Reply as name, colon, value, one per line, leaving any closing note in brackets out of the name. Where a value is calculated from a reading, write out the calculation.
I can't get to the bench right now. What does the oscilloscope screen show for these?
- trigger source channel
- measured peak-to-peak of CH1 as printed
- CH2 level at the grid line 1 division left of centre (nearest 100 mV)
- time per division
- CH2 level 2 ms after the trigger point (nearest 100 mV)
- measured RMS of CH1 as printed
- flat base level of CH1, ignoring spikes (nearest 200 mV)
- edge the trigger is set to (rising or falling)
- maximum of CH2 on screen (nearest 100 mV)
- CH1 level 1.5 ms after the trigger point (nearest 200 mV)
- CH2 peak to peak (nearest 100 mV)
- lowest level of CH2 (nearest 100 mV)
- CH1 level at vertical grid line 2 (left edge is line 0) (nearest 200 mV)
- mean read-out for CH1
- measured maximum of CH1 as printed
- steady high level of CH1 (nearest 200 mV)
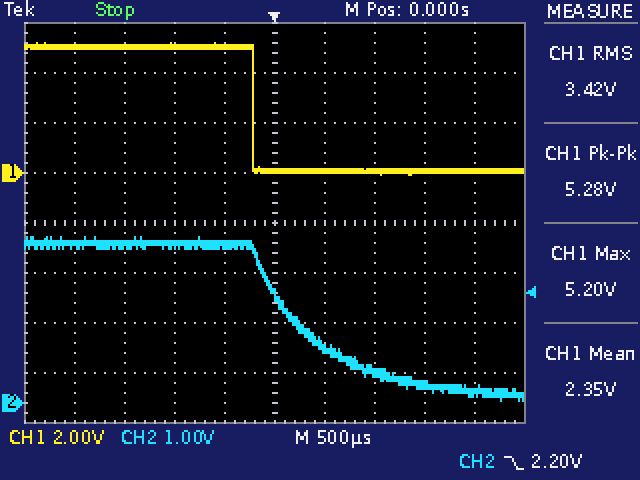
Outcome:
trigger source channel: CH2
measured peak-to-peak of CH1 as printed: 5.28 V
CH2 level at the grid line 1 division left of centre: 3.2 V
time per division: 500 µs
CH2 level 2 ms after the trigger point: 200 mV
measured RMS of CH1 as printed: 3.42 V
flat base level of CH1, ignoring spikes: 0.0 V
edge the trigger is set to: falling
maximum of CH2 on screen: 3.3 V
CH1 level 1.5 ms after the trigger point: 0.0 V
CH2 peak to peak: 3.3 V − (0.0 V) = 3.3 V
lowest level of CH2: 0.0 V
CH1 level at vertical grid line 2 (left edge is line 0): 5.0 V
mean read-out for CH1: 2.35 V
measured maximum of CH1 as printed: 5.20 V
steady high level of CH1: 5.0 V
